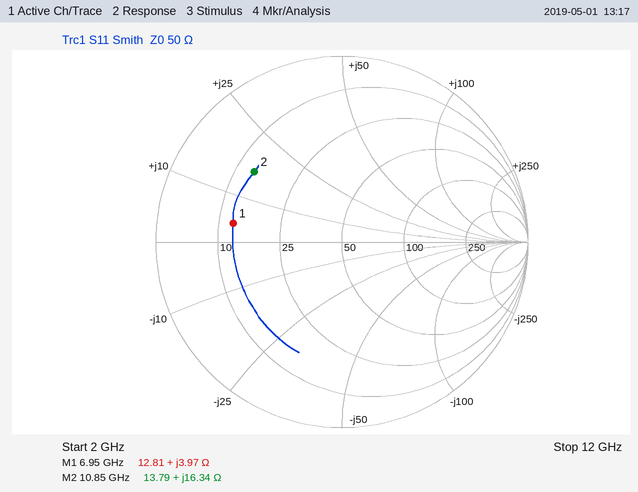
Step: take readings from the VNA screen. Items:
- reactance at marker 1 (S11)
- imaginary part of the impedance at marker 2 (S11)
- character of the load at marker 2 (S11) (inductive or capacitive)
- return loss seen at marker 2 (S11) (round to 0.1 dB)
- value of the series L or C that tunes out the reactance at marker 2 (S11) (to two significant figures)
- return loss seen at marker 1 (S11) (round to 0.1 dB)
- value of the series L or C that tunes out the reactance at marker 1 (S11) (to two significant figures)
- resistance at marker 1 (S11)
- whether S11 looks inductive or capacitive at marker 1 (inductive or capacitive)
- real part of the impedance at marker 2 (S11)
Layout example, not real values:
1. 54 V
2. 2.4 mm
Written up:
1. +3.97 Ω
2. +16.34 Ω
3. inductive
4. 4.4 dB
5. 900 fF
6. 4.5 dB
7. 5.8 pF
8. 12.81 Ω
9. inductive
10. 13.79 Ω
